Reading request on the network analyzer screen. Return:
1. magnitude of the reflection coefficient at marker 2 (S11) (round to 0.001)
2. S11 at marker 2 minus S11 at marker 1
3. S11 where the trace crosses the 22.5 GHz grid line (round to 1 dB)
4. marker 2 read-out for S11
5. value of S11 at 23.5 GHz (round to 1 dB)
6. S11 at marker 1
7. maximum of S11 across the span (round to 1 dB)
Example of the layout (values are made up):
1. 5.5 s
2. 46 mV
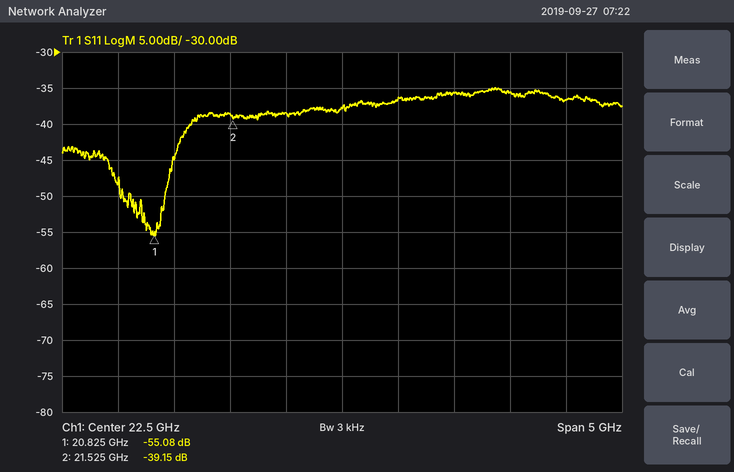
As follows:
1. 0.011
2. 15.93 dB
3. -38 dB
4. -39.15 dB
5. -36 dB
6. -55.08 dB
7. -35 dB
